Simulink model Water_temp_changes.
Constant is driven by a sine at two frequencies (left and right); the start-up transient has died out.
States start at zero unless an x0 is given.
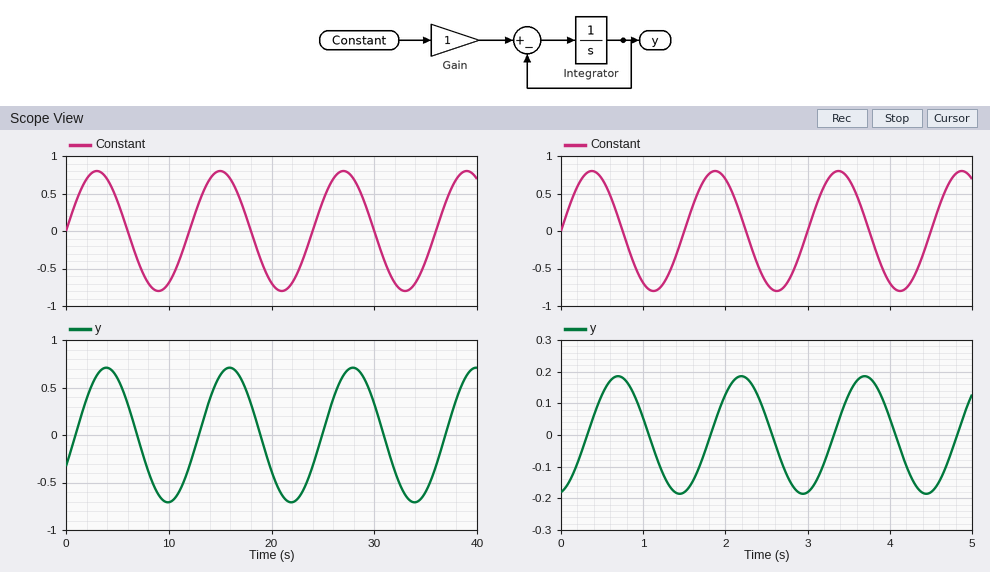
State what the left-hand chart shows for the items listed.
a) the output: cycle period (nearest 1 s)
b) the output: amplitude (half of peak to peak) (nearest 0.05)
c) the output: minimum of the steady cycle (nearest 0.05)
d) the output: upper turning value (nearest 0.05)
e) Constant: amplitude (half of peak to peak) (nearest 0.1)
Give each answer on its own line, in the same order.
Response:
12 s
0.70
-0.70
0.70
0.8
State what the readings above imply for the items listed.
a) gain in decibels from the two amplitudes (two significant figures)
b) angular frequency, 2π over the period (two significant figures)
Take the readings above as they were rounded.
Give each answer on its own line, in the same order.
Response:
-1.2 dB
0.52 rad/s
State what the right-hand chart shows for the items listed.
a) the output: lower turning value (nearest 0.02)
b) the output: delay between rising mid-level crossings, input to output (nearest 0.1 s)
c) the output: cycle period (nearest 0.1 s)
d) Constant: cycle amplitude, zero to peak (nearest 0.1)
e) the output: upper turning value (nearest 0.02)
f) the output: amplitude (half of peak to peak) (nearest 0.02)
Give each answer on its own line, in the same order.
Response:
-0.18
0.3 s
1.5 s
0.8
0.18
0.18
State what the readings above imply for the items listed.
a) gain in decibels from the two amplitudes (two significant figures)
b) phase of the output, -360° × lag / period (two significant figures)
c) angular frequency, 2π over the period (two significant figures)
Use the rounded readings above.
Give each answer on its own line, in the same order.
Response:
-13 dB
-72°
4.2 rad/s
